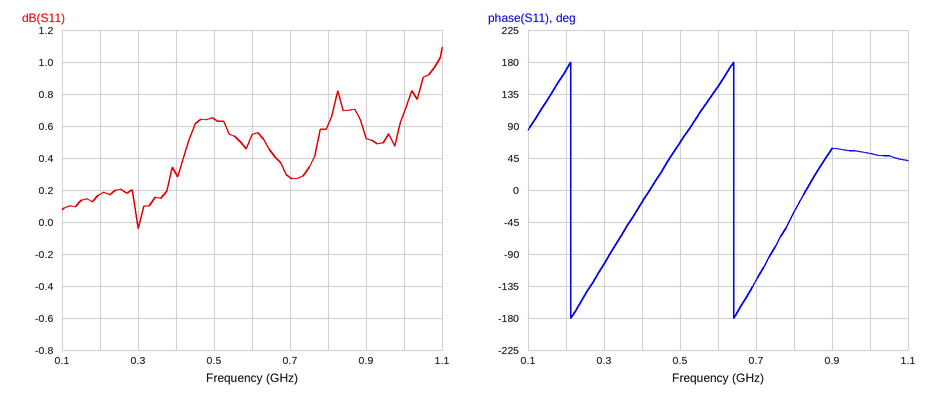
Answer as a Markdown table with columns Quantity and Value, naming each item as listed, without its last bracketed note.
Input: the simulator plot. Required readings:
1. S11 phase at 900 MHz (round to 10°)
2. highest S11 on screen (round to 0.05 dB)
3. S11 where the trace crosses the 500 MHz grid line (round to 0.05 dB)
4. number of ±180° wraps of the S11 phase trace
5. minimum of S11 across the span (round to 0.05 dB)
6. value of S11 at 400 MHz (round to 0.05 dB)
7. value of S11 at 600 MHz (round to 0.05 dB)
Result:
| Quantity | Value |
|---|---|
| S11 phase at 900 MHz | 60° |
| highest S11 on screen | 1.10 dB |
| S11 where the trace crosses the 500 MHz grid line | 0.65 dB |
| number of ±180° wraps of the S11 phase trace | 2 |
| minimum of S11 across the span | -0.05 dB |
| value of S11 at 400 MHz | 0.30 dB |
| value of S11 at 600 MHz | 0.55 dB |
